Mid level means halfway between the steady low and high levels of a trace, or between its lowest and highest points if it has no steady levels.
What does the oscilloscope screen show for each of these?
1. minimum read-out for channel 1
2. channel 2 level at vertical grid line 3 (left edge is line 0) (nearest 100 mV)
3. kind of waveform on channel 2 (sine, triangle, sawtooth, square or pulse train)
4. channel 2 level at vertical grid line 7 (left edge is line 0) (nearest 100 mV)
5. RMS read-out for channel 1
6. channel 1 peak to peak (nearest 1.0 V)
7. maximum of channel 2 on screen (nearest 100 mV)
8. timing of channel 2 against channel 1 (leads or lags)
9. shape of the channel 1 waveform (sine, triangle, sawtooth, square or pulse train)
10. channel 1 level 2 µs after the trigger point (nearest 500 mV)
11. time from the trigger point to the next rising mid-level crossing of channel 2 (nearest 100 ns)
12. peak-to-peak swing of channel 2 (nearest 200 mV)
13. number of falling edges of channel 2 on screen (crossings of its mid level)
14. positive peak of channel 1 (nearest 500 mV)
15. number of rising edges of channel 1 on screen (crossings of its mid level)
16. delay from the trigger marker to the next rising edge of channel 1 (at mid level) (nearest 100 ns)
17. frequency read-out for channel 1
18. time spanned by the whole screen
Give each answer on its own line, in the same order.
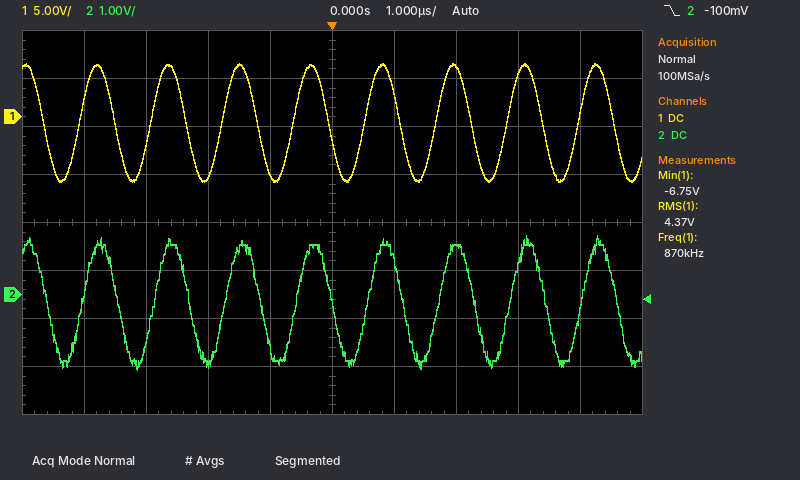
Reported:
-6.75 V
-1.4 V
sine
1.0 V
4.37 V
12.0 V
1.2 V
lags
sine
5.0 V
600 ns
2.8 V
9
5.5 V
8
500 ns
870 kHz
10 µs
